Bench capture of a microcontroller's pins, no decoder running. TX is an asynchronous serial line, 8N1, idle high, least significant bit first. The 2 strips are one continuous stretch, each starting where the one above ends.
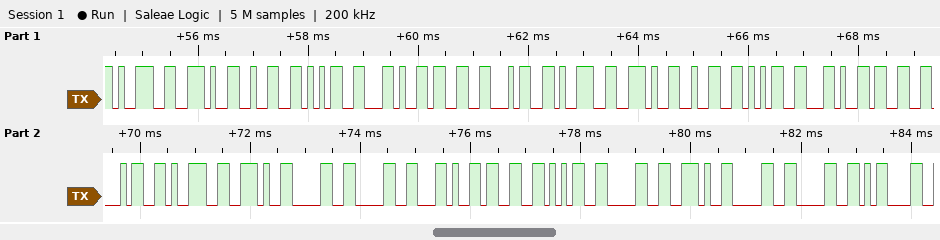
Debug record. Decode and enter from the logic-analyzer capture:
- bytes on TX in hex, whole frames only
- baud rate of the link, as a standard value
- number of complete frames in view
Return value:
0x39 0x2E 0x32 0x35 0x2C 0x33 0x34 0x39 0x2E 0x32 0x35 0x2C 0x33 0x34 0x39 0x2E 0x30 0x30 0x2C 0x33 0x35 0x30 0x2E 0x30 0x30 0x0D
9600 baud
26
